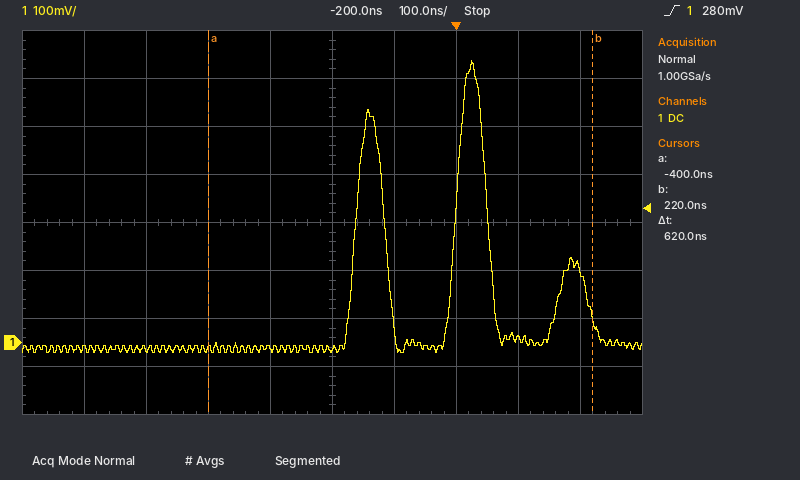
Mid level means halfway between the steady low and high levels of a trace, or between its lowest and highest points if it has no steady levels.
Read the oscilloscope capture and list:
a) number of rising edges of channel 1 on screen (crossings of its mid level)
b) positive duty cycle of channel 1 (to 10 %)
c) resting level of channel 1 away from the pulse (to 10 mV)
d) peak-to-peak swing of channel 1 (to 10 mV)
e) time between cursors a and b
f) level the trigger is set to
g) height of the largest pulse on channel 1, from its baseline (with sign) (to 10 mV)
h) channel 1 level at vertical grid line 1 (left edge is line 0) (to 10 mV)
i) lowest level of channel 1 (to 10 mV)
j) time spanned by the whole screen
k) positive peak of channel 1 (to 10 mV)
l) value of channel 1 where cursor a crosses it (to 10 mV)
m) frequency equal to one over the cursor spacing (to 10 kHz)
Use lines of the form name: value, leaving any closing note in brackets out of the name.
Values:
number of rising edges of channel 1 on screen: 2
positive duty cycle of channel 1: 30 %
resting level of channel 1 away from the pulse: -10 mV
peak-to-peak swing of channel 1: 610 mV
time between cursors a and b: 620 ns
level the trigger is set to: 280 mV
height of the largest pulse on channel 1, from its baseline (with sign): +600 mV
channel 1 level at vertical grid line 1 (left edge is line 0): -10 mV
lowest level of channel 1: -20 mV
time spanned by the whole screen: 1 µs
positive peak of channel 1: 590 mV
value of channel 1 where cursor a crosses it: -10 mV
frequency equal to one over the cursor spacing: 1.61 MHz
